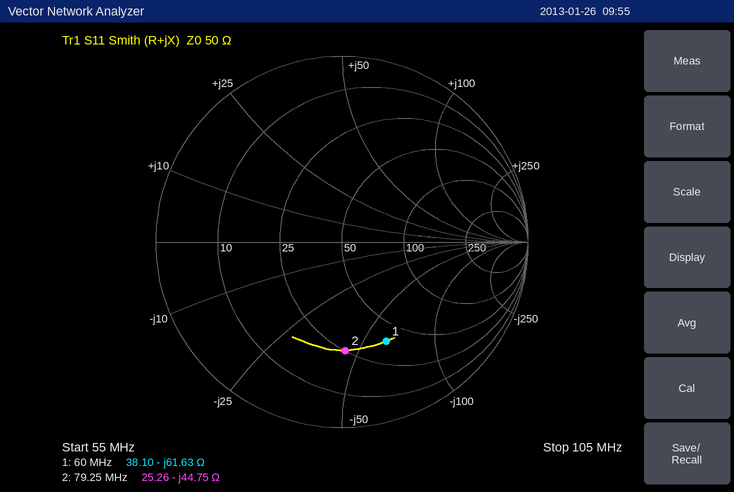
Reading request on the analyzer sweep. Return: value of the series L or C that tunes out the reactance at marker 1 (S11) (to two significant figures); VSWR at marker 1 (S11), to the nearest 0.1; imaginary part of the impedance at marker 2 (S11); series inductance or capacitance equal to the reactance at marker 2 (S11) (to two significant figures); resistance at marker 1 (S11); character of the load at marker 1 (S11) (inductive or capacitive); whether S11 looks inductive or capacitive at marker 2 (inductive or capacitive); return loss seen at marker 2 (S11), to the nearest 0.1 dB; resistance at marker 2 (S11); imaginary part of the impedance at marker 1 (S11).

160 nH
3.8
-44.75 Ω
45 pF
38.10 Ω
capacitive
capacitive
4.7 dB
25.26 Ω
-61.63 Ω
